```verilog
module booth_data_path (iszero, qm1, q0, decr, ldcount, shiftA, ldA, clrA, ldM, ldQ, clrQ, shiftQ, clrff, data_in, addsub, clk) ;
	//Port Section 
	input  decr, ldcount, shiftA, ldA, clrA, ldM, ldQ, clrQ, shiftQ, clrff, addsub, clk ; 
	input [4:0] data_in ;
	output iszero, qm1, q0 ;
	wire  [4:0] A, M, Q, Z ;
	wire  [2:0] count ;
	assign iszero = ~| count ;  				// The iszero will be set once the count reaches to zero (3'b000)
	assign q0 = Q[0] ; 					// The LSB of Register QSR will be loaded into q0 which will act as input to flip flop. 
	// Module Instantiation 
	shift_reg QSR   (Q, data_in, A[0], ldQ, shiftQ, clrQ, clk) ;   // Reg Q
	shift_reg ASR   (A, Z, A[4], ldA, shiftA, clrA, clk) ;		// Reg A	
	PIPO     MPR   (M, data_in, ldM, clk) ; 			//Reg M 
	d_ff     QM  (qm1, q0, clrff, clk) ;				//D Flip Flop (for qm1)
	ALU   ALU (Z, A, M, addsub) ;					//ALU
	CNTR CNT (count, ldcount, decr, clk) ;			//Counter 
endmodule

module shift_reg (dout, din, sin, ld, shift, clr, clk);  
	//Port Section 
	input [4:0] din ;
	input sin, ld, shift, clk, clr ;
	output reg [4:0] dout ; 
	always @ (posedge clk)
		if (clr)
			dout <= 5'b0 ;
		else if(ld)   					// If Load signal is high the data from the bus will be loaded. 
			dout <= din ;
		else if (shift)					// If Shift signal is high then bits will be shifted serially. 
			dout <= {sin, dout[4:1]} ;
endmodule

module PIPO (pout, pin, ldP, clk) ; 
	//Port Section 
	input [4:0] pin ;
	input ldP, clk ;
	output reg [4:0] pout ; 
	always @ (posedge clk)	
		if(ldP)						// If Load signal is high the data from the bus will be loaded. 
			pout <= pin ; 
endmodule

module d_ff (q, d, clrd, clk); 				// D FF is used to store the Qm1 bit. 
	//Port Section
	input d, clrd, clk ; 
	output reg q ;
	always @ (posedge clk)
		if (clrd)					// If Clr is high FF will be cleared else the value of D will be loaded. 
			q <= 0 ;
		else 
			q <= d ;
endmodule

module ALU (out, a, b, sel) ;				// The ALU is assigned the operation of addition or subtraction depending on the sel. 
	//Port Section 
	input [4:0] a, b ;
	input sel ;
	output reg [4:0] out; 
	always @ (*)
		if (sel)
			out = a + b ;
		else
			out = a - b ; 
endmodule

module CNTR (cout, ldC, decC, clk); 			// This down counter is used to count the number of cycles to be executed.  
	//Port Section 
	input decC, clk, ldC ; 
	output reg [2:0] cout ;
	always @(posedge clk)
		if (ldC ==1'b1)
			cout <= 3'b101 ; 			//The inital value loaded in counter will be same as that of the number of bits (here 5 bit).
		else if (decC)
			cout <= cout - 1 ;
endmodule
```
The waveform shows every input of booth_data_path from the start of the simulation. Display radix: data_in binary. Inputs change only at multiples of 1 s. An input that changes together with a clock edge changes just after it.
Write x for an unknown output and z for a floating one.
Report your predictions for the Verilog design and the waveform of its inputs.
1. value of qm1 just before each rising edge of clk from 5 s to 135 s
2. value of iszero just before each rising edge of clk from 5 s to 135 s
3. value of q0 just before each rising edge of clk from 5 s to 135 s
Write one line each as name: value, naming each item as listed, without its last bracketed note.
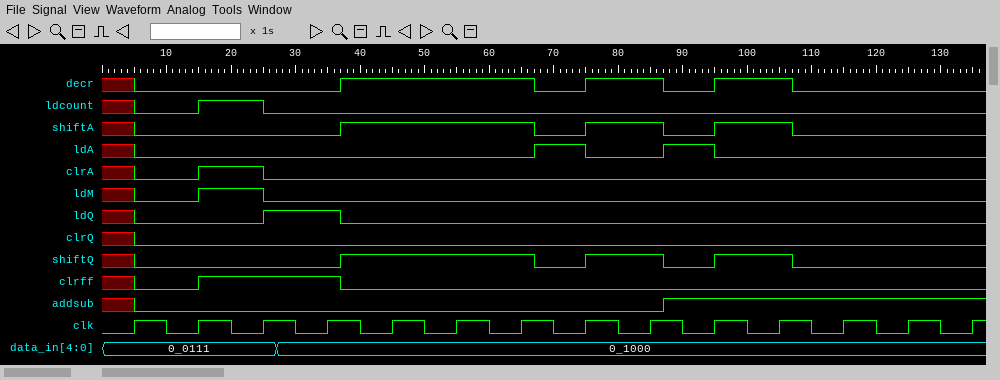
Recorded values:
value of qm1 just before each rising edge of clk from 5 s to 135 s: x x x 0 0 0 0 0 1 1 0 0 0 0
value of iszero just before each rising edge of clk from 5 s to 135 s: x x x 0 0 0 0 0 0 0 0 1 1 1
value of q0 just before each rising edge of clk from 5 s to 135 s: x x x x 0 0 0 1 1 0 0 0 0 0
